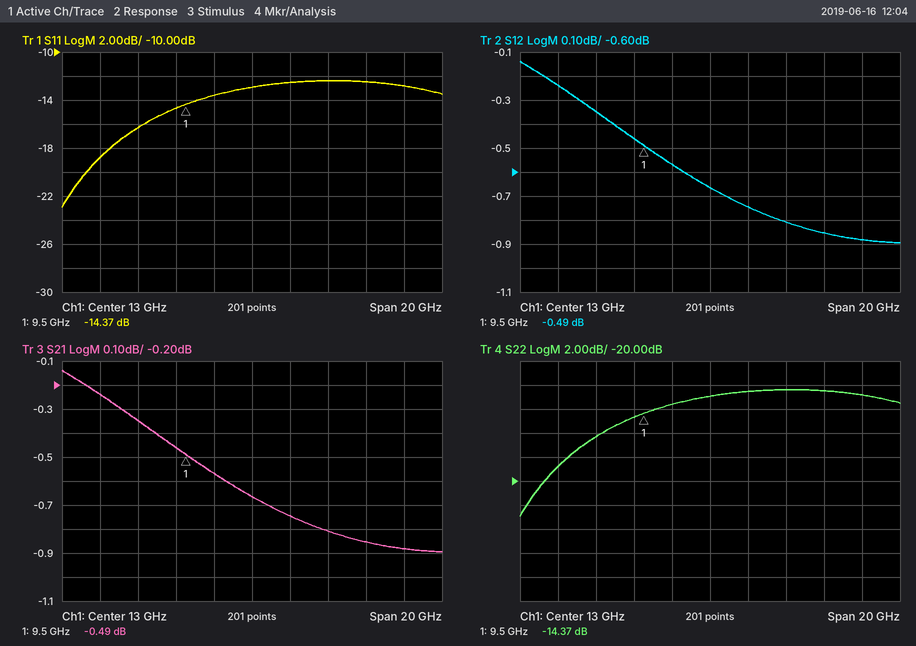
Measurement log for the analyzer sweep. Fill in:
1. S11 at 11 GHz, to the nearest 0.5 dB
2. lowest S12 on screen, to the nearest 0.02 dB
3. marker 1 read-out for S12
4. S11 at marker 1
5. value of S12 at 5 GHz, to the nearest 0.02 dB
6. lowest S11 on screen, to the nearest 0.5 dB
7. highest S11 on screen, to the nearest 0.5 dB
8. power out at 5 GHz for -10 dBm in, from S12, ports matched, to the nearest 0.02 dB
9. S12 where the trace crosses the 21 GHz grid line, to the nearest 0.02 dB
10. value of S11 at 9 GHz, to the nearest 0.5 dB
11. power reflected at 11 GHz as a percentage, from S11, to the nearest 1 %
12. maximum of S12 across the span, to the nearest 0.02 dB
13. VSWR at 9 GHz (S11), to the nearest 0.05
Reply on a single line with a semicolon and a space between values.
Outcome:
-13.5 dB; -0.90 dB; -0.49 dB; -14.37 dB; -0.24 dB; -23.0 dB; -12.5 dB; -10.24 dBm; -0.88 dB; -14.5 dB; 4 %; -0.14 dB; 1.45
